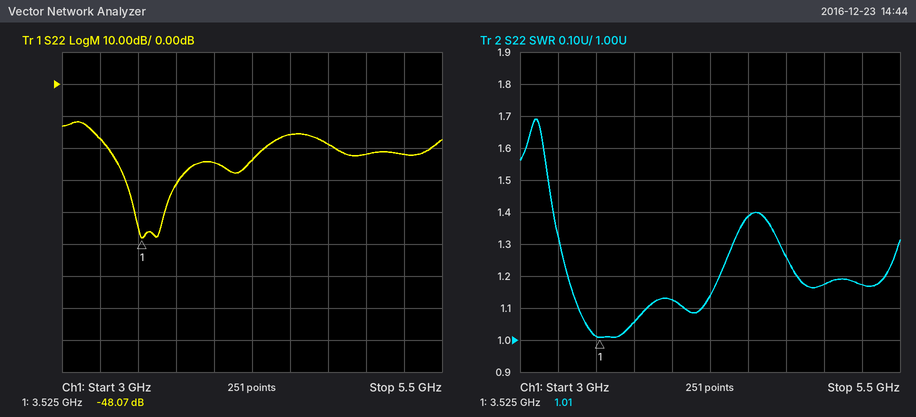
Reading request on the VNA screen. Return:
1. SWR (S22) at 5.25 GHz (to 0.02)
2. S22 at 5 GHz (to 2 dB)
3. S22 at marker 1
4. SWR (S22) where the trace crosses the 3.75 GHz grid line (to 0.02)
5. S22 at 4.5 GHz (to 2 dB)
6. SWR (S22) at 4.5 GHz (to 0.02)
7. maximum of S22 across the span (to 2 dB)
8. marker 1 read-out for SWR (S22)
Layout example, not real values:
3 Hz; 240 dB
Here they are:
1.18; -22 dB; -48.07 dB; 1.06; -16 dB; 1.38; -12 dB; 1.01
